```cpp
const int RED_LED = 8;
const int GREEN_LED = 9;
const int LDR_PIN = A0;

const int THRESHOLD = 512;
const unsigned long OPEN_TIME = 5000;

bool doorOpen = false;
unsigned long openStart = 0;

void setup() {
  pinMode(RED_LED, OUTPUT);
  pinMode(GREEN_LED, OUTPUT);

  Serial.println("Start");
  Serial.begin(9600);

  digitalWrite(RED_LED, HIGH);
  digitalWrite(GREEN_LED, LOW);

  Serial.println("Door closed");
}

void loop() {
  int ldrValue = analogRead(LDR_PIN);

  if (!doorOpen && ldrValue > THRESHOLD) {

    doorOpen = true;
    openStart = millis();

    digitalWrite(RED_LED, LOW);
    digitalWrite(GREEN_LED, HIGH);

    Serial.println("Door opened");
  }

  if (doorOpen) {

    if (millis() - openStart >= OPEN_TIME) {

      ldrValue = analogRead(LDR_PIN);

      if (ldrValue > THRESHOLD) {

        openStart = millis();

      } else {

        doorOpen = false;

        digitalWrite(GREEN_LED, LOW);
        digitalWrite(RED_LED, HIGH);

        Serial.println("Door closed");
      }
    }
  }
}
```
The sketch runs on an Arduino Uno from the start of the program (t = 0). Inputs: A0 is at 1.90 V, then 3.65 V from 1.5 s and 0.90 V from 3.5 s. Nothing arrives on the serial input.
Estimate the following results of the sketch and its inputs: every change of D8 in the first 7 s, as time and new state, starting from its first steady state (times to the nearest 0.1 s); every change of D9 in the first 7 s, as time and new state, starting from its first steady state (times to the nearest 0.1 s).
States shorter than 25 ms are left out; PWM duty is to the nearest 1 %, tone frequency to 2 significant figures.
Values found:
0 s high; 1.5 s low; 6.5 s high
0 s low; 1.5 s high; 6.5 s low
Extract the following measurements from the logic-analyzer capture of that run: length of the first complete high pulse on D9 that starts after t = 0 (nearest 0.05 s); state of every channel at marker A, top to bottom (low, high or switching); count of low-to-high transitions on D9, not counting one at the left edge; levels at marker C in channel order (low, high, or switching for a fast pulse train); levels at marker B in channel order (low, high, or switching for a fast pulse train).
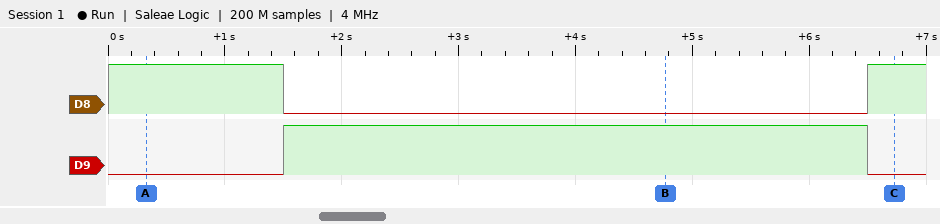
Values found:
5.00 s
D8 high, D9 low
1
D8 high, D9 low
D8 low, D9 high
